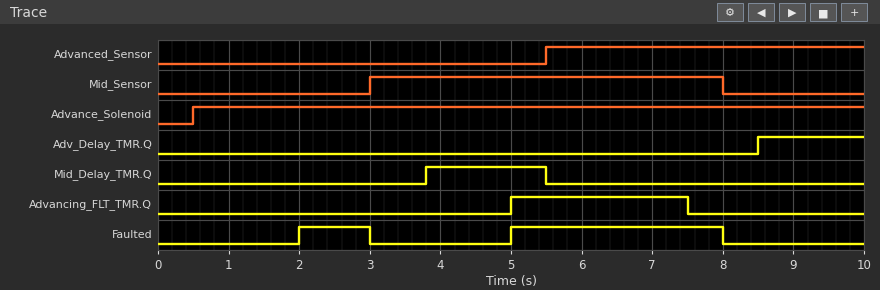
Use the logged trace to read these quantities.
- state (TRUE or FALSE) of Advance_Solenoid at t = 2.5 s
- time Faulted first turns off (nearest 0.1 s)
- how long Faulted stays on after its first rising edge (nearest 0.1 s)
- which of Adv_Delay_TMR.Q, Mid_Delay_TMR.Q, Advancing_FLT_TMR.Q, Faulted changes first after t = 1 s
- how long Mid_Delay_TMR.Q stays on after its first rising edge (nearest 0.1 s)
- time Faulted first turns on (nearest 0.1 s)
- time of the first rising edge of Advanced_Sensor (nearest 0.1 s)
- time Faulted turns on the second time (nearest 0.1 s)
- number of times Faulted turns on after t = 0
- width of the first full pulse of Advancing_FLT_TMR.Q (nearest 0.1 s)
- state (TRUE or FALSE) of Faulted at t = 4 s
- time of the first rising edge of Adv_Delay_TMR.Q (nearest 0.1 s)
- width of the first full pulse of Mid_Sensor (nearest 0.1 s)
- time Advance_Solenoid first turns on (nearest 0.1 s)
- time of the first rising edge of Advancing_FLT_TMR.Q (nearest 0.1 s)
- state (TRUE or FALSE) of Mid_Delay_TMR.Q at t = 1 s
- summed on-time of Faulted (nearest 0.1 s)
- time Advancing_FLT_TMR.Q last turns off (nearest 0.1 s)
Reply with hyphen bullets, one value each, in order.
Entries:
- TRUE
- 3.0 s
- 1.0 s
- Faulted
- 1.7 s
- 2.0 s
- 5.5 s
- 5.0 s
- 2
- 2.5 s
- FALSE
- 8.5 s
- 5.0 s
- 0.5 s
- 5.0 s
- FALSE
- 4.0 s
- 7.5 s
